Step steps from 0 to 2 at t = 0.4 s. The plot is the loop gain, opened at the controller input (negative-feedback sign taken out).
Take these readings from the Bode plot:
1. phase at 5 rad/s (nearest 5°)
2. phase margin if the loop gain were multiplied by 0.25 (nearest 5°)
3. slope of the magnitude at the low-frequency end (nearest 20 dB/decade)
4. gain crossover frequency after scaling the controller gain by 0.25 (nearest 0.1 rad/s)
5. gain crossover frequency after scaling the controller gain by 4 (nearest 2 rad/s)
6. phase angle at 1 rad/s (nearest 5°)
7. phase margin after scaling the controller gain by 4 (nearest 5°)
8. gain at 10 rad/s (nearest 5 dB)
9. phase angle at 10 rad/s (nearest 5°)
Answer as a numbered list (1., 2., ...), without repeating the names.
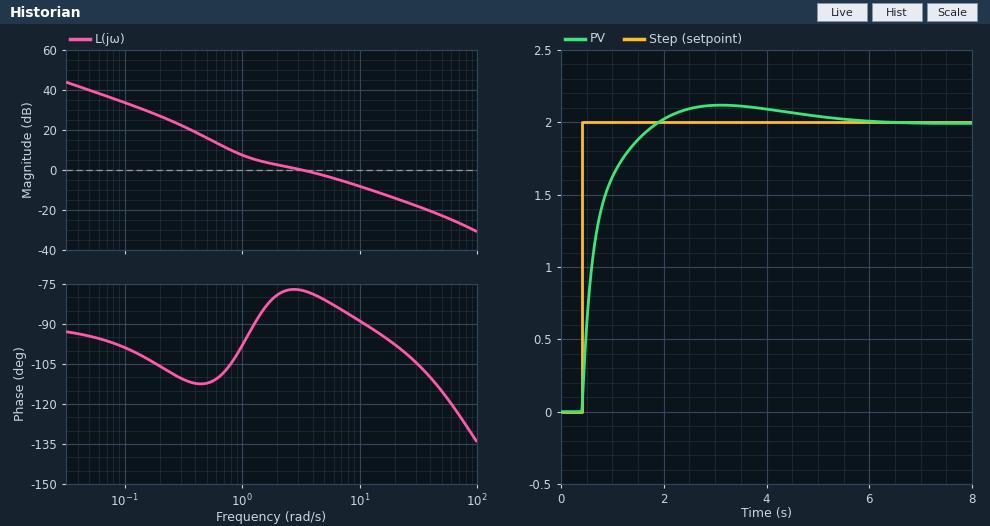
1. -80°
2. 70°
3. -20 dB/decade
4. 0.7 rad/s
5. 16 rad/s
6. -100°
7. 85°
8. -10 dB
9. -90°
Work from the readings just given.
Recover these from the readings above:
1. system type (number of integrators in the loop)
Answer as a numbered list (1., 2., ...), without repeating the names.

1. 1
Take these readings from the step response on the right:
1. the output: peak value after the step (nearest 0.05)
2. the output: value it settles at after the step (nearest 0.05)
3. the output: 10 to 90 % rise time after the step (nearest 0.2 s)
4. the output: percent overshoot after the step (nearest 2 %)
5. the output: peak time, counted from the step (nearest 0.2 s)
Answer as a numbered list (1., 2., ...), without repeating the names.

1. 2.10
2. 2.00
3. 0.8 s
4. 6 %
5. 2.8 s
